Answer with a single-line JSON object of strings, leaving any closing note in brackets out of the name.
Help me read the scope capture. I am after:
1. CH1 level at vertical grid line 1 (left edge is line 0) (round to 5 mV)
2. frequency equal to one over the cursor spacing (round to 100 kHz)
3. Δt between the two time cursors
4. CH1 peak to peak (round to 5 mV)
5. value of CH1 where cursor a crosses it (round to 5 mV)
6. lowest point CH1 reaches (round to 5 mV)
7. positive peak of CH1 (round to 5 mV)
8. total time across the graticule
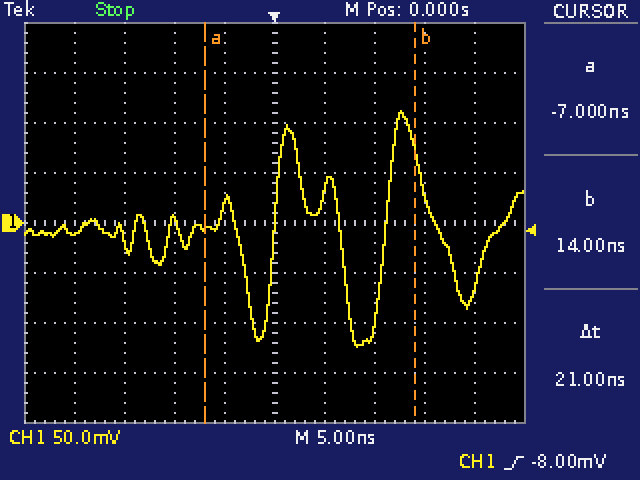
{"CH1 level at vertical grid line 1 (left edge is line 0)": "-10 mV", "frequency equal to one over the cursor spacing": "47.6 MHz", "Δt between the two time cursors": "21 ns", "CH1 peak to peak": "235 mV", "value of CH1 where cursor a crosses it": "-5 mV", "lowest point CH1 reaches": "-125 mV", "positive peak of CH1": "110 mV", "total time across the graticule": "50 ns"}
